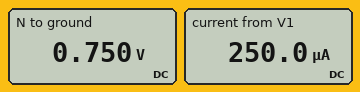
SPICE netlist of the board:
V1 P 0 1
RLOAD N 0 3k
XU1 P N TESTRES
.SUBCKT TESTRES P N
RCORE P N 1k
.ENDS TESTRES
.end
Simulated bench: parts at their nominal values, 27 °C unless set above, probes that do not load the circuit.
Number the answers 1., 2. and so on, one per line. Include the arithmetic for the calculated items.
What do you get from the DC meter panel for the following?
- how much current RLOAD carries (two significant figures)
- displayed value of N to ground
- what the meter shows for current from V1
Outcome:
1. (750 mV) / 3 kΩ = 250 µA
2. 0.750 V
3. 250.0 µA
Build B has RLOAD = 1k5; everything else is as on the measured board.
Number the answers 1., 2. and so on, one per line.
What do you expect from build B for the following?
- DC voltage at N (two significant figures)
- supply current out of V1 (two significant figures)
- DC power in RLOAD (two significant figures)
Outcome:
1. 600 mV
2. 400 µA
3. 240 µW
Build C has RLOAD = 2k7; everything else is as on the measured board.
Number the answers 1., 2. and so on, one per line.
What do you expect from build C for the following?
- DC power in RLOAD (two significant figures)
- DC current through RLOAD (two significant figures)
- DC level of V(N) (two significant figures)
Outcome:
1. 200 µW
2. 270 µA
3. 730 mV
